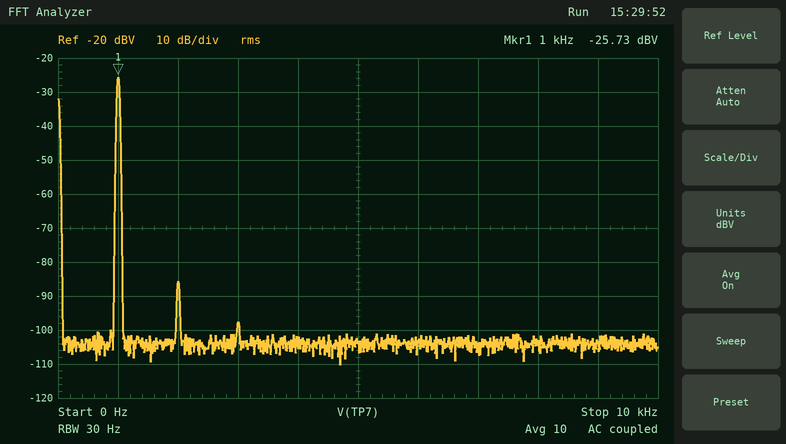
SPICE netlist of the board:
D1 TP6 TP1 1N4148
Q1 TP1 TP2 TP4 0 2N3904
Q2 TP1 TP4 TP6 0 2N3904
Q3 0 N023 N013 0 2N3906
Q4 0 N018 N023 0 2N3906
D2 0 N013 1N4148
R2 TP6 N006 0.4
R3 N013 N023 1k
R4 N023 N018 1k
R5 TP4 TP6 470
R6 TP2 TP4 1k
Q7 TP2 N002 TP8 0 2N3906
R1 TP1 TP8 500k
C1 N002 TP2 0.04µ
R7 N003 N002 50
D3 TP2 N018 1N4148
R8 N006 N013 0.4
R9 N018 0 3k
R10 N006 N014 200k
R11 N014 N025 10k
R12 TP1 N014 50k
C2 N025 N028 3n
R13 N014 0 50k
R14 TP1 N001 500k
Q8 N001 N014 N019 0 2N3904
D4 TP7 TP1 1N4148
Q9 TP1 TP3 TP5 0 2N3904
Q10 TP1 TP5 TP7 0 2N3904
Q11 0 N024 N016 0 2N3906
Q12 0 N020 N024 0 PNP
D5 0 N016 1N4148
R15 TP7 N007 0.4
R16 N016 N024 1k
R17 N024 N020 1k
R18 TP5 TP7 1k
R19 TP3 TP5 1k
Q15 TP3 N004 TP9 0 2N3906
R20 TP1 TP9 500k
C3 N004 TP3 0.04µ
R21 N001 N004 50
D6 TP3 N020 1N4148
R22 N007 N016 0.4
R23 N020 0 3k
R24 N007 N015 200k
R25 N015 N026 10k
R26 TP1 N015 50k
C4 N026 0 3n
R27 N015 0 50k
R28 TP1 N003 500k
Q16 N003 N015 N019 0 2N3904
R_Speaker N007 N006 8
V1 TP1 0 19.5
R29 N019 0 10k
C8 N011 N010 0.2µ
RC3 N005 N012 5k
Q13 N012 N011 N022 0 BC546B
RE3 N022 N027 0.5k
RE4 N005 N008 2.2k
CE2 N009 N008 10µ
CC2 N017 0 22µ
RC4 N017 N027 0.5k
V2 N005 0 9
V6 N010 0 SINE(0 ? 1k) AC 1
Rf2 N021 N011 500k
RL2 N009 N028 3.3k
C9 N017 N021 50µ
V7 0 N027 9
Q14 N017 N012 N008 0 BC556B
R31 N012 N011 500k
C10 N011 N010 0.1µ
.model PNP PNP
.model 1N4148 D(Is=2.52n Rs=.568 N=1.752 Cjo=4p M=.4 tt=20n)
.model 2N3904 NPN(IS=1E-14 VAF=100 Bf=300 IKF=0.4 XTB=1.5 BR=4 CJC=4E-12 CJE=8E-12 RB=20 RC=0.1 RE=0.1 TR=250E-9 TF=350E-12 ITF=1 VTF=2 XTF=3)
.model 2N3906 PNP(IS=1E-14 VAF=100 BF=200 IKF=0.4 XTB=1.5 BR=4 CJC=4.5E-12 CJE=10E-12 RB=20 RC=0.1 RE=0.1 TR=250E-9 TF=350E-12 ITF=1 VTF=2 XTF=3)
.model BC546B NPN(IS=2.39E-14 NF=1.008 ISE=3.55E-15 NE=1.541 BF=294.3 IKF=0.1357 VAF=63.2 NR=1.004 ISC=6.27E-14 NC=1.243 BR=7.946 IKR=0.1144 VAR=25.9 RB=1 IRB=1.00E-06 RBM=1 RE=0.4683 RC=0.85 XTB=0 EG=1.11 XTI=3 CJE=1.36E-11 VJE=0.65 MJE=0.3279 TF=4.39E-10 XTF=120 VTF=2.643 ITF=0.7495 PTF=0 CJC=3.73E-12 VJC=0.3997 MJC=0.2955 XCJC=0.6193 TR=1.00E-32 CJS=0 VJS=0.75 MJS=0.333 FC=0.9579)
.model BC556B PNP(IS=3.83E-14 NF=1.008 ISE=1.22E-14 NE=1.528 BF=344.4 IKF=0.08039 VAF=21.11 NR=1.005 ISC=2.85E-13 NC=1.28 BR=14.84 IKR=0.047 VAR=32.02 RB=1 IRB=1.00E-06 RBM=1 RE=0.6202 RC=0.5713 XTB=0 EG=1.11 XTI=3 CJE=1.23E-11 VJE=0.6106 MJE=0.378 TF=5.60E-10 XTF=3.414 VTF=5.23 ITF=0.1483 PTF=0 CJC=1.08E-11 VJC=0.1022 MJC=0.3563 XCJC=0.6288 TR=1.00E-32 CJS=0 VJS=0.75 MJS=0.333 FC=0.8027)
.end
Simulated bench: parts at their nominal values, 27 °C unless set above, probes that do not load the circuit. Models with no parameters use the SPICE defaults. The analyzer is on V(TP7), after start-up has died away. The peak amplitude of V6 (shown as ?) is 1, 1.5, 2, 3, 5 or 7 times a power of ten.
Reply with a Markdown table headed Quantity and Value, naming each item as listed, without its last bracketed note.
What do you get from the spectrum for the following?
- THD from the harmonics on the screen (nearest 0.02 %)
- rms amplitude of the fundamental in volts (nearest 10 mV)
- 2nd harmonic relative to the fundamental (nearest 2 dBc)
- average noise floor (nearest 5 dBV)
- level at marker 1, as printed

| Quantity | Value |
|---|---|
| THD from the harmonics on the screen | 0.10 % |
| rms amplitude of the fundamental in volts | 50 mV |
| 2nd harmonic relative to the fundamental | -60 dBc |
| average noise floor | -105 dBV |
| level at marker 1, as printed | -25.73 dBV |
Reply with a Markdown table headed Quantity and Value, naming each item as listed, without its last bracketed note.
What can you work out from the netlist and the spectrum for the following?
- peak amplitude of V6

| Quantity | Value |
|---|---|
| peak amplitude of V6 | 300 mV |
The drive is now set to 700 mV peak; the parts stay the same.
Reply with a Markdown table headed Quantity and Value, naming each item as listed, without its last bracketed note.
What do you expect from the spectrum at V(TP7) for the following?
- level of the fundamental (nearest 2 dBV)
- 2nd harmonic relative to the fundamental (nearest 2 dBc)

| Quantity | Value |
|---|---|
| level of the fundamental | -18 dBV |
| 2nd harmonic relative to the fundamental | -38 dBc |
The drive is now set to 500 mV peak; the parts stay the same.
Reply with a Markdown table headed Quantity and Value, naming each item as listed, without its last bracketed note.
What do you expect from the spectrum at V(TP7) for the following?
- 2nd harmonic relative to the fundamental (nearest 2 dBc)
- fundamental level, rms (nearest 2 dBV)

| Quantity | Value |
|---|---|
| 2nd harmonic relative to the fundamental | -16 dBc |
| fundamental level, rms | -22 dBV |
